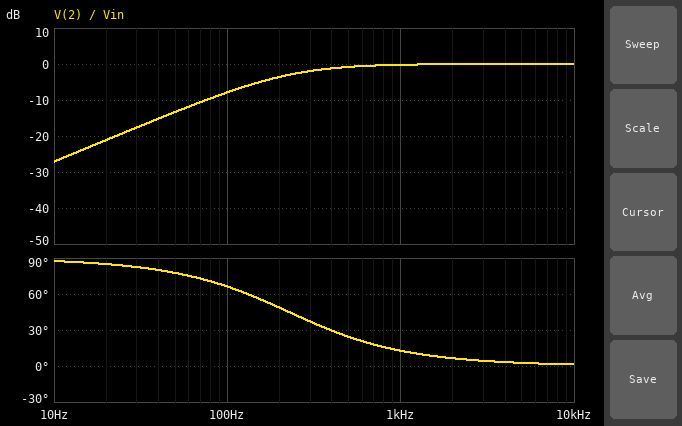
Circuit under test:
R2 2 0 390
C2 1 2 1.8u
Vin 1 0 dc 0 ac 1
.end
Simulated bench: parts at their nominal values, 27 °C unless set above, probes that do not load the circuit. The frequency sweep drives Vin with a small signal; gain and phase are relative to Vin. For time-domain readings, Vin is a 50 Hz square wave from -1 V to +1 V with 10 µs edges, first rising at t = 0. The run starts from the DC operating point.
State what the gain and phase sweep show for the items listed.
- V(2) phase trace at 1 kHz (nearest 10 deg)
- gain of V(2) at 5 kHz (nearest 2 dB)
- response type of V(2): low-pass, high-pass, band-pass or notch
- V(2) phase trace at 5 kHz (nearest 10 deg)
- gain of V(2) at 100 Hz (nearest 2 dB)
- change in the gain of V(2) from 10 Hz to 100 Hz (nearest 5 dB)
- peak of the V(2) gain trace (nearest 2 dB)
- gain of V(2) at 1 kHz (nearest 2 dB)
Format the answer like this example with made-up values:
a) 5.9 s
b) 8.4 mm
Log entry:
a) 10 deg
b) 0 dB
c) high-pass
d) 0 deg
e) -8 dB
f) 20 dB
g) 0 dB
h) 0 dB
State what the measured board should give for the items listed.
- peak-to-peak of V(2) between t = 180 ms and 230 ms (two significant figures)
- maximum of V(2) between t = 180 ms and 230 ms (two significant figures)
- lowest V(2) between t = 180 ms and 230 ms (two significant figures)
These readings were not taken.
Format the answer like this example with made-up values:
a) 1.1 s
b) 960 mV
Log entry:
a) 4.0 V
b) 2.0 V
c) -2.0 V
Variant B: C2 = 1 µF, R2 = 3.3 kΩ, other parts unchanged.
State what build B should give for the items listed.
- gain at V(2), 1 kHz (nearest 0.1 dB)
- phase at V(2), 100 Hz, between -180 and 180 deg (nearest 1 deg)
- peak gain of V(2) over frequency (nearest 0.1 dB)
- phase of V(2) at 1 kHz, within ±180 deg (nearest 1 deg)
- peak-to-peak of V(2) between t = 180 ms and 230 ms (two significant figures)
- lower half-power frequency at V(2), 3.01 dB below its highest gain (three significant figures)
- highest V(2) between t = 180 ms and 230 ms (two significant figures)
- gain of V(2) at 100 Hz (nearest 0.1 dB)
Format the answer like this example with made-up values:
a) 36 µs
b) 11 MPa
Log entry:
a) 0 dB
b) 26 deg
c) 0 dB
d) 3 deg
e) 3.8 V
f) 48.2 Hz
g) 1.9 V
h) -0.9 dB
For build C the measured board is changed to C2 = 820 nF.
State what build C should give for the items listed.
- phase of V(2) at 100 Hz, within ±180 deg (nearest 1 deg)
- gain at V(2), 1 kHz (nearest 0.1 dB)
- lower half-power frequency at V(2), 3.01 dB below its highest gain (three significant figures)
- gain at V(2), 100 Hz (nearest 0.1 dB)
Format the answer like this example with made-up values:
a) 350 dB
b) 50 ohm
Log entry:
a) 79 deg
b) -1.0 dB
c) 498 Hz
d) -14.1 dB
